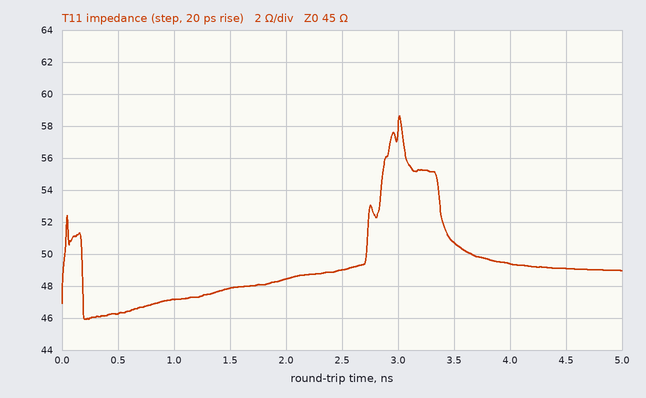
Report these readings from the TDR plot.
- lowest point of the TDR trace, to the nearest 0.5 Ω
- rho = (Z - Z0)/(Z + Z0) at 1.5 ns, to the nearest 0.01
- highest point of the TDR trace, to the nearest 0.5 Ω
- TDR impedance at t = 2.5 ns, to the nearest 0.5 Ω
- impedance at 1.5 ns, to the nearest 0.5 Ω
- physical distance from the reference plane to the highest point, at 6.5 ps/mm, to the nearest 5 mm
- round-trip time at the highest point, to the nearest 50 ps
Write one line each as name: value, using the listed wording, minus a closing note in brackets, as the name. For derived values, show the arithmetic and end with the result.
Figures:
lowest point of the TDR trace, to the nearest 0.5 Ω: 46.0 Ω
rho = (Z - Z0)/(Z + Z0) at 1.5 ns, to the nearest 0.01: (48 − 45)/(48 + 45) ≈ +0.03
highest point of the TDR trace, to the nearest 0.5 Ω: 58.5 Ω
TDR impedance at t = 2.5 ns, to the nearest 0.5 Ω: 49.0 Ω
impedance at 1.5 ns, to the nearest 0.5 Ω: 48.0 Ω
physical distance from the reference plane to the highest point, at 6.5 ps/mm, to the nearest 5 mm: 3.00 ns / 2 / 6.5 ps/mm ≈ 231 mm, so 230 mm to the nearest 5 mm
round-trip time at the highest point, to the nearest 50 ps: 3.00 ns
